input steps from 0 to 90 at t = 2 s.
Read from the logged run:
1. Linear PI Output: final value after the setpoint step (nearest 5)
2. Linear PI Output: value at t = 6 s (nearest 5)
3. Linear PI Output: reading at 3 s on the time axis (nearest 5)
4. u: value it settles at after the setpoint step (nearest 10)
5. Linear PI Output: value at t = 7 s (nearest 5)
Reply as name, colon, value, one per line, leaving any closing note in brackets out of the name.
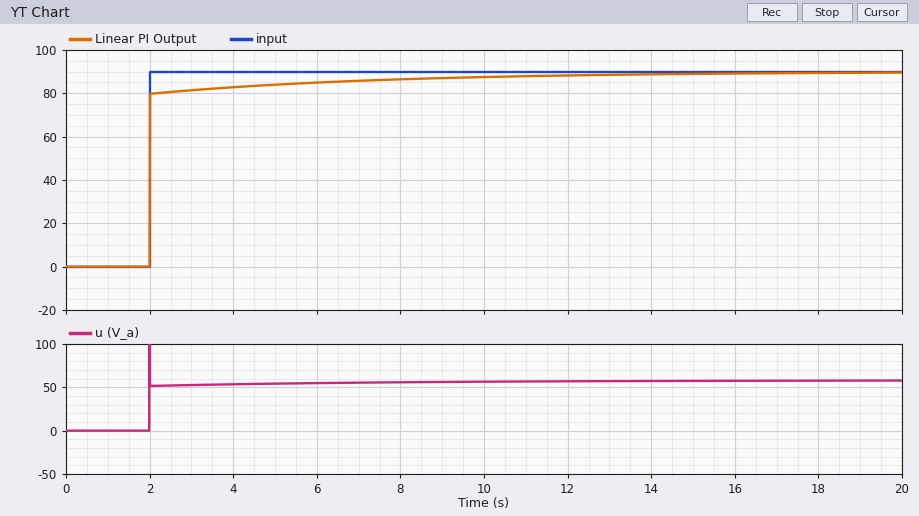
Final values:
Linear PI Output: final value after the setpoint step: 90
Linear PI Output: value at t = 6 s: 85
Linear PI Output: reading at 3 s on the time axis: 80
u: value it settles at after the setpoint step: 60
Linear PI Output: value at t = 7 s: 85
